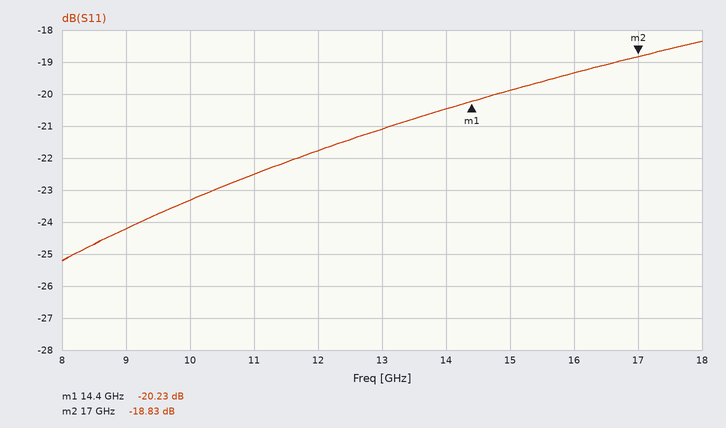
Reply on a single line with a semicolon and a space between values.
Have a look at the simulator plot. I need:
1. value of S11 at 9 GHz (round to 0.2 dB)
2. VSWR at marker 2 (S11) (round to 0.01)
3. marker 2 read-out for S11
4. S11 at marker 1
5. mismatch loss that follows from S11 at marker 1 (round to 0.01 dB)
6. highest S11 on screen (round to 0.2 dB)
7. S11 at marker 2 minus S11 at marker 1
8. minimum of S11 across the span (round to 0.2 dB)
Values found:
-24.2 dB; 1.26; -18.83 dB; -20.23 dB; 0.04 dB; -18.4 dB; 1.40 dB; -25.2 dB
